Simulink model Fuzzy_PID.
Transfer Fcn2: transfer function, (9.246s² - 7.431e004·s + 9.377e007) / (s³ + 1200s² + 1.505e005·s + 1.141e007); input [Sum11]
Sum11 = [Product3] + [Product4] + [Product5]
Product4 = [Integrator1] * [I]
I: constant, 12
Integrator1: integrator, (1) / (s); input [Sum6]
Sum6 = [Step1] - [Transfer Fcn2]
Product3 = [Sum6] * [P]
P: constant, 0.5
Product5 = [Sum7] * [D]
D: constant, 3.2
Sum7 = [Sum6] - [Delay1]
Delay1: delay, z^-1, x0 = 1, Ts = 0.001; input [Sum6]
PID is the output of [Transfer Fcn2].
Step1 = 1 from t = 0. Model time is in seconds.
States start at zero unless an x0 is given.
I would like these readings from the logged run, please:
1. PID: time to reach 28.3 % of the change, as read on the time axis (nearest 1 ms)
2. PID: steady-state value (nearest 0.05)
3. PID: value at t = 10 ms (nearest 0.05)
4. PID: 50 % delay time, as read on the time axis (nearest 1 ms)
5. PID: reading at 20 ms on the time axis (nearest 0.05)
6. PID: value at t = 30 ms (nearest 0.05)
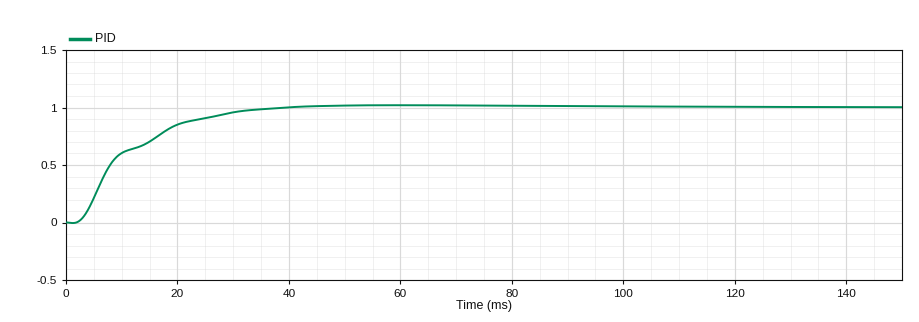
6 ms
1.00
0.60
8 ms
0.85
0.95
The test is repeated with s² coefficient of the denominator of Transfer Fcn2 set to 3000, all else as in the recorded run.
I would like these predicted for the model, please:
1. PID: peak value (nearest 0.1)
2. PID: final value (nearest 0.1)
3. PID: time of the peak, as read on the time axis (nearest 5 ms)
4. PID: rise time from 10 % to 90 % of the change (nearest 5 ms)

1.0
1.0
35 ms
15 ms
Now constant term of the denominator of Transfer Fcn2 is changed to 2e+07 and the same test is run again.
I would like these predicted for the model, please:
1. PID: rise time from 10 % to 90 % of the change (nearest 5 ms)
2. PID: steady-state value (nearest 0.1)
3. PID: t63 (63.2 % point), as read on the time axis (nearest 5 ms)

35 ms
1.0
15 ms
